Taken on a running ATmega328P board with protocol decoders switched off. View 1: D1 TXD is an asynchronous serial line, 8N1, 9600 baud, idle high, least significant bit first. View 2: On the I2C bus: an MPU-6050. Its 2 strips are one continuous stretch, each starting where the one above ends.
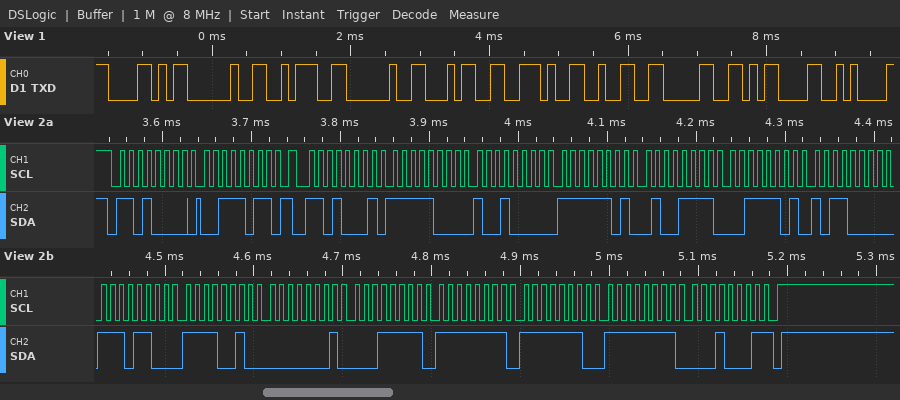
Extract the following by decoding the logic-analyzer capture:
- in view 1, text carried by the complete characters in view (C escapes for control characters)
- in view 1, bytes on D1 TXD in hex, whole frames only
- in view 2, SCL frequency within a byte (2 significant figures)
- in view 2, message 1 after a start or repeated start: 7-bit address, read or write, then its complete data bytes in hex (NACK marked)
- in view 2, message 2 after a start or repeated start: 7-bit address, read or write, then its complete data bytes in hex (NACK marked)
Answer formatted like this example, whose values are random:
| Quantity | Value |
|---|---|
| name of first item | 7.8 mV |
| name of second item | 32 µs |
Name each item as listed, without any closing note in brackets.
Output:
| Quantity | Value |
|---|---|
| in view 1, text carried by the complete characters in view | "X : 4.20\r\n" |
| in view 1, bytes on D1 TXD in hex, whole frames only | 58 20 3A 20 34 2E 32 30 0D 0A |
| in view 2, SCL frequency within a byte | 100 kHz |
| in view 2, message 1 after a start or repeated start: 7-bit address, read or write, then its complete data bytes in hex | 0x68 write: 3B |
| in view 2, message 2 after a start or repeated start: 7-bit address, read or write, then its complete data bytes in hex | 0x68 read: F8 90 FD 4F 3D B0 EC F2 01 1F FF FE FF 11 NACK |
